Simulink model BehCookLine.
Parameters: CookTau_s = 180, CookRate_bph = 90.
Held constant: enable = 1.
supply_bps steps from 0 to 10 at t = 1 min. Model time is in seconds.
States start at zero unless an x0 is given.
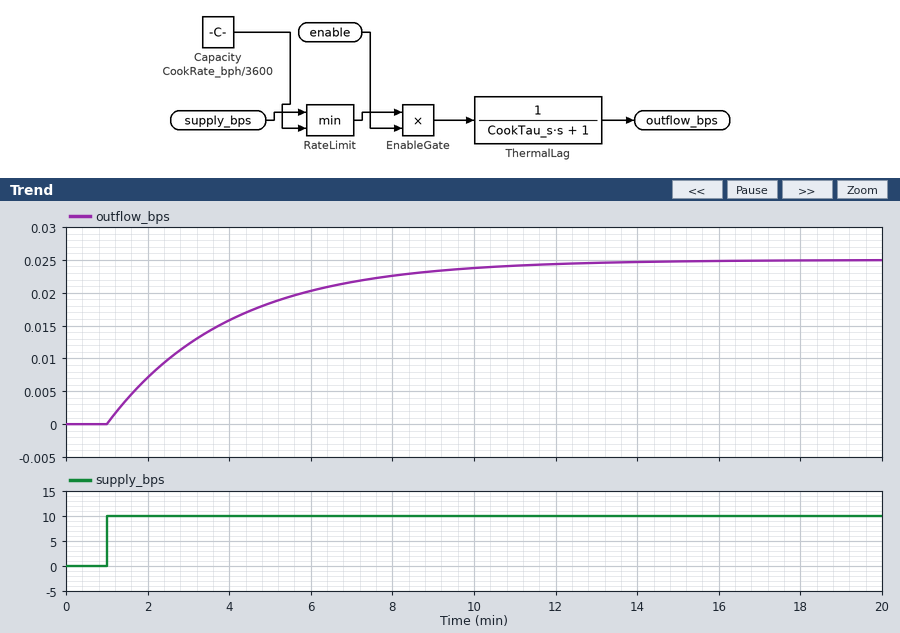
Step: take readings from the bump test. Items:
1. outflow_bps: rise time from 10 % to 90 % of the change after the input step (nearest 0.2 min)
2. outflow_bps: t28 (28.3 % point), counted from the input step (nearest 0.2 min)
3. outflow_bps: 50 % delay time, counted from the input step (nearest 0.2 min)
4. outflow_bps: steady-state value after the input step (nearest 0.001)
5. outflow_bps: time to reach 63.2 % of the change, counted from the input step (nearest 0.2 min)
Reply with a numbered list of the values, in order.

1. 6.6 min
2. 1.0 min
3. 2.0 min
4. 0.025
5. 3.0 min
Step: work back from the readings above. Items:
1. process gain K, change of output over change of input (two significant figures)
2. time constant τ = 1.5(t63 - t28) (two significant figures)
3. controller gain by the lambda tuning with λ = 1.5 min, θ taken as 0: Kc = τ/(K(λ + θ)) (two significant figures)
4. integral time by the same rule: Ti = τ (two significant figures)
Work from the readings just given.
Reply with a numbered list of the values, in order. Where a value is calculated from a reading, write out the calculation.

1. (0.025 - 0) / 10 = 0.0025
2. 1.5 × (3 - 1) = 3.0 min
3. 3 / (0.0025 × (1.5 + 0)) = 800
4. 3.0 min
